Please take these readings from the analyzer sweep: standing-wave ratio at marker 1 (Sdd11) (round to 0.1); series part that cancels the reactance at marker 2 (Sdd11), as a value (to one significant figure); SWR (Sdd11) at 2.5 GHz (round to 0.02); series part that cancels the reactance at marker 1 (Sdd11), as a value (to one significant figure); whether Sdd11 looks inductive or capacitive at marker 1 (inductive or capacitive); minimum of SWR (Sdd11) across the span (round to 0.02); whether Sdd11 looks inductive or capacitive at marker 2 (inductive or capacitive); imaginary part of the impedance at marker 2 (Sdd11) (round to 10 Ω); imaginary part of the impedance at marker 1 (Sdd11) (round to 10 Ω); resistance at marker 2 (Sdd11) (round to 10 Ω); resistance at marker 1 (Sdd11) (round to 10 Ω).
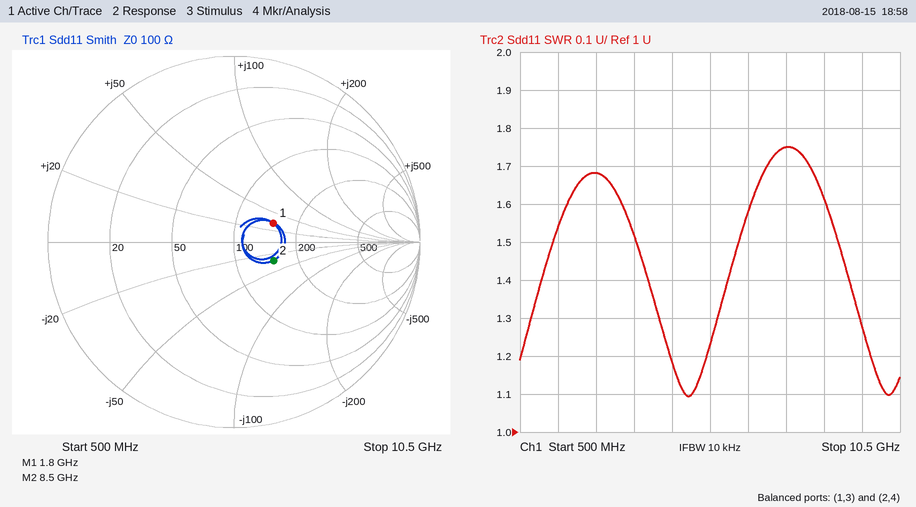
1.6
600 pH
1.68
3 pF
inductive
1.10
capacitive
-30 Ω
+30 Ω
150 Ω
150 Ω
